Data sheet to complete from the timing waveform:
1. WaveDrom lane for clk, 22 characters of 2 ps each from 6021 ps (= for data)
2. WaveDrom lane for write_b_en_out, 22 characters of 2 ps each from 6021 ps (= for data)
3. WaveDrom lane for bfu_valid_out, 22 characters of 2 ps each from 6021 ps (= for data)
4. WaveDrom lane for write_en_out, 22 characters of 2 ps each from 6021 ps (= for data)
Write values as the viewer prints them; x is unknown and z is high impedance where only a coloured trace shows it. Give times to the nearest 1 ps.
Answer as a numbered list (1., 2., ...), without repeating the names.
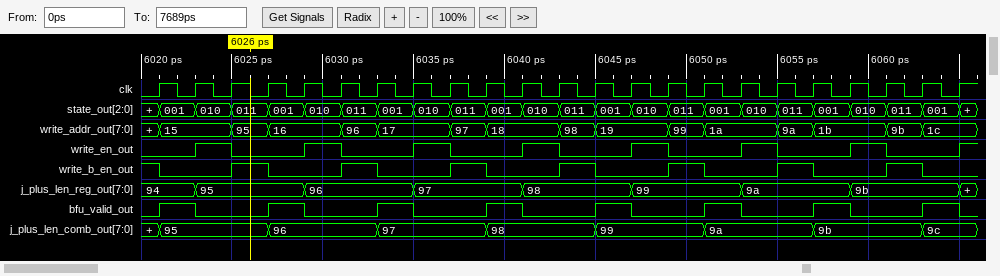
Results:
1. {name: 'clk', wave: 'p.....................'}
2. {name: 'write_b_en_out', wave: '0.10.10.10.10.10.10.10'}
3. {name: 'bfu_valid_out', wave: '10.10.10.10.10.10.10.1'}
4. {name: 'write_en_out', wave: '010.10.10.10.10.10.10.'}
